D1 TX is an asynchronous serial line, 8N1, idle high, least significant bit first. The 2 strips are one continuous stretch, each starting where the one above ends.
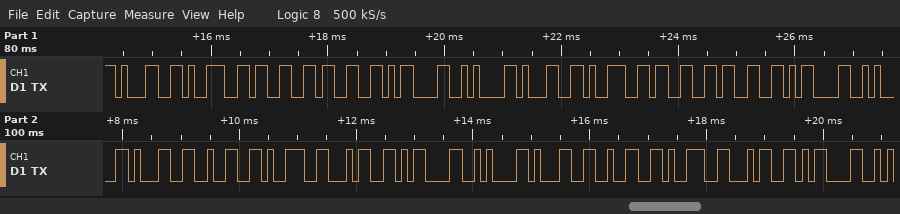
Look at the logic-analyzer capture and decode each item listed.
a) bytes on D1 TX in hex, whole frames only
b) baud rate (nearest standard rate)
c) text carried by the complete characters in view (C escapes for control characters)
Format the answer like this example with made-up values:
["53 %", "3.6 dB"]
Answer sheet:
["31 39 33 33 0D 0A 31 39 33 33 0D 0A 31 32 39 34 0D 0A 31 32 39 34 0D", "9600 baud", "\"1933\\r\\n1933\\r\\n1294\\r\\n1294\\r\""]
